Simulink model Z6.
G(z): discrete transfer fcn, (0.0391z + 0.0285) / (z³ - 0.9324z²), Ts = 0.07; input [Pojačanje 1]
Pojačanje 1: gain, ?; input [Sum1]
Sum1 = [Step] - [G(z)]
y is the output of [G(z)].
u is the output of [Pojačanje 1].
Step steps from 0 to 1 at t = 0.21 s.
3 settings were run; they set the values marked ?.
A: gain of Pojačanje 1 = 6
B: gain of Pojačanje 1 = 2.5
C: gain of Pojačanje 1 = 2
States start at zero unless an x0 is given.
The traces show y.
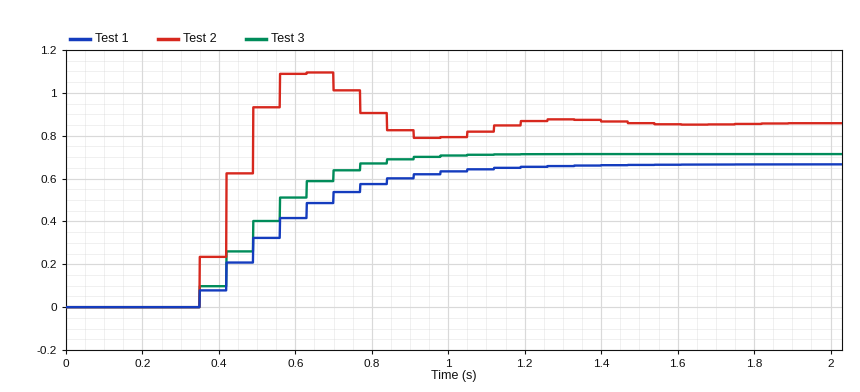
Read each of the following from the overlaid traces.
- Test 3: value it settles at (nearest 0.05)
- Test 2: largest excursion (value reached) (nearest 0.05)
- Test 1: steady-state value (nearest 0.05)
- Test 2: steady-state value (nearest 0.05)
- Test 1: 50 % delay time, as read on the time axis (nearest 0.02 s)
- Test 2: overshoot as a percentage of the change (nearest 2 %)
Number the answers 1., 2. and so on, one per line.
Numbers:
1. 0.70
2. 1.10
3. 0.65
4. 0.85
5. 0.56 s
6. 28 %
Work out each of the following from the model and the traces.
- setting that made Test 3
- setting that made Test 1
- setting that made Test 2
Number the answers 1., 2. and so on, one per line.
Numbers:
1. B
2. C
3. A
